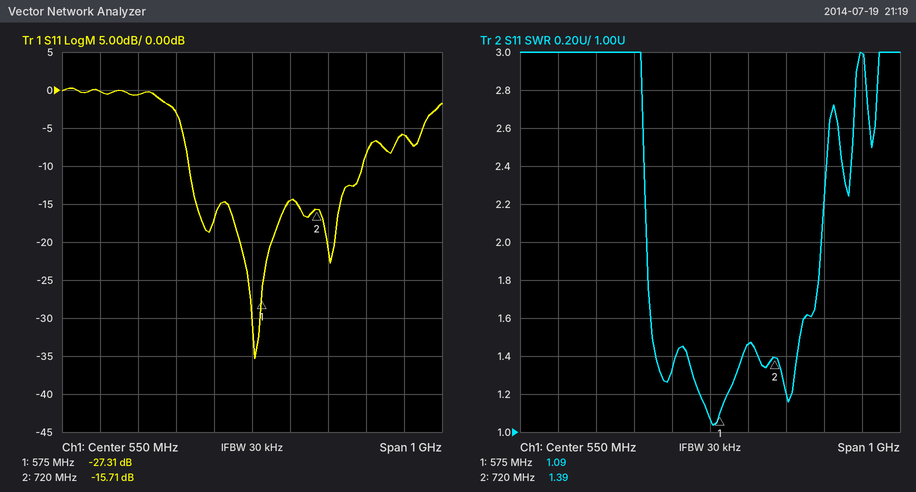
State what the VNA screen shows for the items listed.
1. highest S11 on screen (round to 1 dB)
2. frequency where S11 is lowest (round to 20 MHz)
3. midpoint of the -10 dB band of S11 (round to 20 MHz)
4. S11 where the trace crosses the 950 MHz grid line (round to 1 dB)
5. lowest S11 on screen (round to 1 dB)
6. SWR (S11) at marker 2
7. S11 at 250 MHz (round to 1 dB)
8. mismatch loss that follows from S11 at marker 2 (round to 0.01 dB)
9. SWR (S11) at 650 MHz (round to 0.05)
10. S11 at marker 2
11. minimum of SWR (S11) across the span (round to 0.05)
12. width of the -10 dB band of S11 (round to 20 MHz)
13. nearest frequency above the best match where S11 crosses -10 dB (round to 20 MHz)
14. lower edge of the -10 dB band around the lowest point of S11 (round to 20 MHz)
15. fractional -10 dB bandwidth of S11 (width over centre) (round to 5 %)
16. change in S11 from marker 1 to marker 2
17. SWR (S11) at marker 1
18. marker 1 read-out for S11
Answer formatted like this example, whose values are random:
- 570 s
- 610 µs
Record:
- 0 dB
- 560 MHz
- 620 MHz
- -6 dB
- -35 dB
- 1.39
- -1 dB
- 0.12 dB
- 1.45
- -15.71 dB
- 1.05
- 460 MHz
- 840 MHz
- 380 MHz
- 75 %
- 11.60 dB
- 1.09
- -27.31 dB
